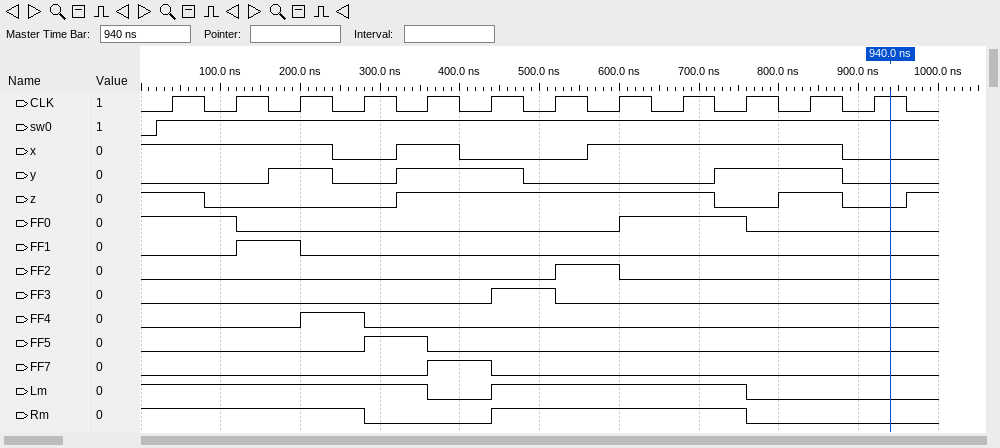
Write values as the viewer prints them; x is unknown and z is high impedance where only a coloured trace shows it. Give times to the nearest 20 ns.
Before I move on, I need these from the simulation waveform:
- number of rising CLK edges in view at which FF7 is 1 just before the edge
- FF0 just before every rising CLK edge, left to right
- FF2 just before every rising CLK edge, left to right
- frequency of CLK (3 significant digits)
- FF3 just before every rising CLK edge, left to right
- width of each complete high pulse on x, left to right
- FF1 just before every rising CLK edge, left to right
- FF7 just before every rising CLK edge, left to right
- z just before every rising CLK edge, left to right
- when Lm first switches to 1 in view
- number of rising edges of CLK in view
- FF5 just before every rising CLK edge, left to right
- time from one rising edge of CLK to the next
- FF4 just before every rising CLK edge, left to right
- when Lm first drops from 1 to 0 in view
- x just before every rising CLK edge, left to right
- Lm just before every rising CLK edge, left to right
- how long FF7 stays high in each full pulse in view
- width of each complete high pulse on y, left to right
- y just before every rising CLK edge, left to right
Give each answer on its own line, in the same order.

1
1 1 0 0 0 0 0 0 1 1 0 0
0 0 0 0 0 0 0 1 0 0 0 0
12.5 MHz
0 0 0 0 0 0 1 0 0 0 0 0
80 ns, 320 ns
0 0 1 0 0 0 0 0 0 0 0 0
0 0 0 0 0 1 0 0 0 0 0 0
1 0 0 0 1 1 1 1 1 0 1 0
440 ns
12
0 0 0 0 1 0 0 0 0 0 0 0
80 ns
0 0 0 1 0 0 0 0 0 0 0 0
360 ns
1 1 1 0 1 0 0 1 1 1 1 0
1 1 1 1 1 0 1 1 1 1 0 0
80 ns
80 ns, 160 ns, 160 ns
0 0 1 0 1 1 0 0 0 1 1 0
